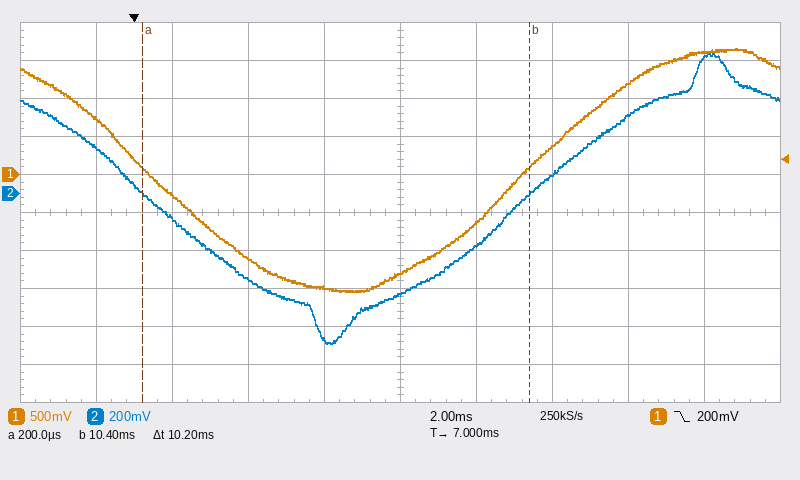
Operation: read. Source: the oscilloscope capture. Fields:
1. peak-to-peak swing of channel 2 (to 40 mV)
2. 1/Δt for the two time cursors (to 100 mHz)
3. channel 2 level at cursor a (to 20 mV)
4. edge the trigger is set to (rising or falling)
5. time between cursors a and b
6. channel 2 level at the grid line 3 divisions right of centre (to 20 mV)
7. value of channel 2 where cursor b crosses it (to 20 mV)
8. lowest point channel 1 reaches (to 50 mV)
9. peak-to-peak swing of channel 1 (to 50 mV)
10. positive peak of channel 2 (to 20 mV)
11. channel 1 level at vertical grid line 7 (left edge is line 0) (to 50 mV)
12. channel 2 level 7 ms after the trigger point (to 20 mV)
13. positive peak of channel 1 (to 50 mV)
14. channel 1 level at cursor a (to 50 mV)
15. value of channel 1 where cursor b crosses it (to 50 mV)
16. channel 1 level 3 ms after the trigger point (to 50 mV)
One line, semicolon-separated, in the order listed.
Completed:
1.52 V; 98.0 Hz; 0 mV; falling; 10.2 ms; 400 mV; 0 mV; -1.55 V; 3.20 V; 740 mV; 350 mV; -540 mV; 1.65 V; 100 mV; 100 mV; -1.10 V
